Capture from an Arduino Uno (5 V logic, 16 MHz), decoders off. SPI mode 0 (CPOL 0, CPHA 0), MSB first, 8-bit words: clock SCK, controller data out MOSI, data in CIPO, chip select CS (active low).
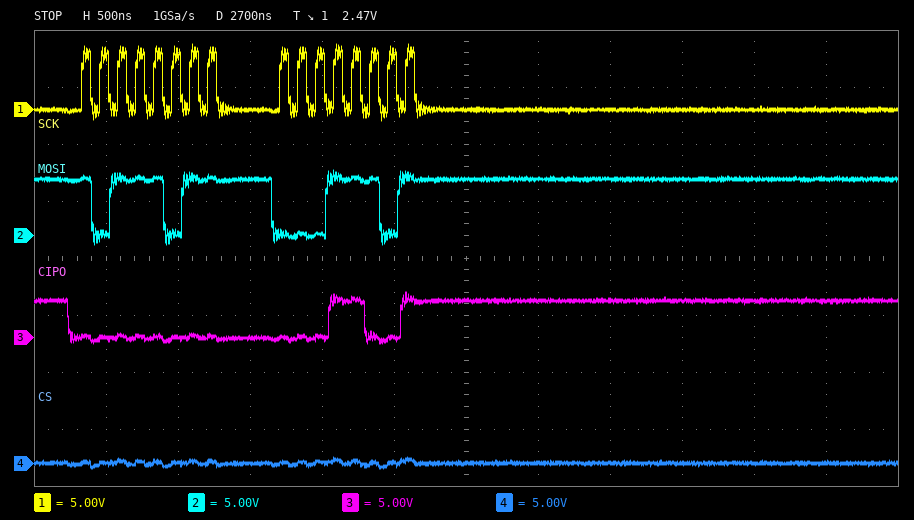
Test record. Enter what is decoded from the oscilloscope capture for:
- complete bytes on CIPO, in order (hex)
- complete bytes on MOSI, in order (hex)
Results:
0x00 0x19
0xBB 0x1D
